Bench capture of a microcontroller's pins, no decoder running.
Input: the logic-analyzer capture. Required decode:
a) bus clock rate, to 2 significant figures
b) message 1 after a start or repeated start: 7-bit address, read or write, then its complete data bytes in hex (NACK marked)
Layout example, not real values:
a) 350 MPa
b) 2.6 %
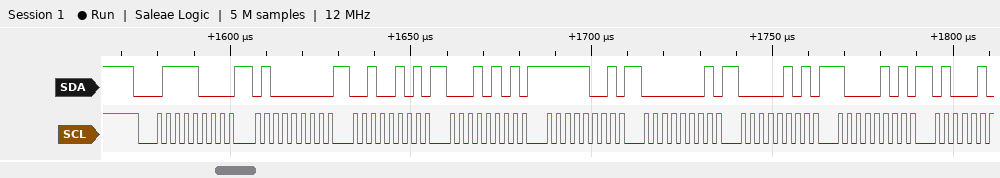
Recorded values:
a) 400 kHz
b) 0x3C write: 40 25 15 F9 01 05 85
